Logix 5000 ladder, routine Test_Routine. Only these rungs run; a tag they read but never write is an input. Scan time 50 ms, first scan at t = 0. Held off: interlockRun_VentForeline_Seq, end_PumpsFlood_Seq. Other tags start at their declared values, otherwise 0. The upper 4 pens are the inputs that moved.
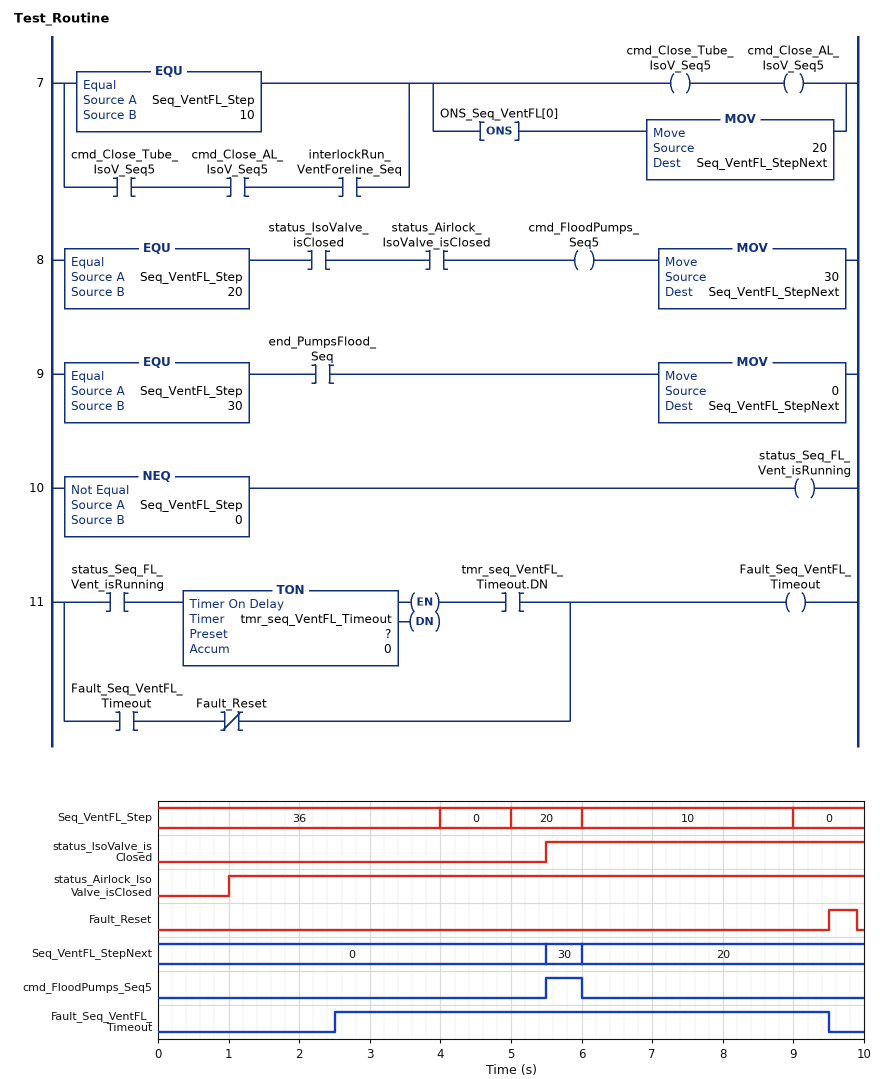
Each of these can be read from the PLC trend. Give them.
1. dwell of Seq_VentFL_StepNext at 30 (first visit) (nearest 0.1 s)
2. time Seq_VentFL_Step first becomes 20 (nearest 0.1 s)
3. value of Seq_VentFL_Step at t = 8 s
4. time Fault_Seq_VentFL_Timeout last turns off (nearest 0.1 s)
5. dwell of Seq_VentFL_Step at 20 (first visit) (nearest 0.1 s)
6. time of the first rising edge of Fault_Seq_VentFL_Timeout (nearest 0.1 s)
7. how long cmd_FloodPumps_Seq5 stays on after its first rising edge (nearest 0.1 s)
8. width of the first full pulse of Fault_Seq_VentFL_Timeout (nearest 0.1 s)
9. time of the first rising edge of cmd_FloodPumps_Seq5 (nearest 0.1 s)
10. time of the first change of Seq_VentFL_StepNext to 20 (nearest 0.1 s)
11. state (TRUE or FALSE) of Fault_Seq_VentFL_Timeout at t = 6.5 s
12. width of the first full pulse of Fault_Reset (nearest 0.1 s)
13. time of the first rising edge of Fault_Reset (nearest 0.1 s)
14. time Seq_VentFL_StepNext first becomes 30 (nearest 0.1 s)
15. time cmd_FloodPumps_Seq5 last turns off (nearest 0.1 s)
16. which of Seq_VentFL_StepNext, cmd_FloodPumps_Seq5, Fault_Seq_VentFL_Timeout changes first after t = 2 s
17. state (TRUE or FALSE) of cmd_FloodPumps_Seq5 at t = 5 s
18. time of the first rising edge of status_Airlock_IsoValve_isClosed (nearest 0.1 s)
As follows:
0.5 s
5.0 s
10
9.5 s
1.0 s
2.5 s
0.5 s
7.0 s
5.5 s
6.0 s
TRUE
0.4 s
9.5 s
5.5 s
6.0 s
Fault_Seq_VentFL_Timeout
FALSE
1.0 s
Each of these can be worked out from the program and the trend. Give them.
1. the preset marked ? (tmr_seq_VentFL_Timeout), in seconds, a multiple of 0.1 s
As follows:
2.5 s
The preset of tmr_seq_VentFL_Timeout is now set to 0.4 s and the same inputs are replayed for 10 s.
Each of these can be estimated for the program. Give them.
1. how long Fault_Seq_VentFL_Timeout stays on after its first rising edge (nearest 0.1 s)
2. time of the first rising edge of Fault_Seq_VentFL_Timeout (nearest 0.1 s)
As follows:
9.1 s
0.4 s
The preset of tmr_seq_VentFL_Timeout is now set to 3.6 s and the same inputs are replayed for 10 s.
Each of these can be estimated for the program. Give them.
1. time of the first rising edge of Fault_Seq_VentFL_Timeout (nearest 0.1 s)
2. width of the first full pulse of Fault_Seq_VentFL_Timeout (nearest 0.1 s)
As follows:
3.6 s
5.9 s
